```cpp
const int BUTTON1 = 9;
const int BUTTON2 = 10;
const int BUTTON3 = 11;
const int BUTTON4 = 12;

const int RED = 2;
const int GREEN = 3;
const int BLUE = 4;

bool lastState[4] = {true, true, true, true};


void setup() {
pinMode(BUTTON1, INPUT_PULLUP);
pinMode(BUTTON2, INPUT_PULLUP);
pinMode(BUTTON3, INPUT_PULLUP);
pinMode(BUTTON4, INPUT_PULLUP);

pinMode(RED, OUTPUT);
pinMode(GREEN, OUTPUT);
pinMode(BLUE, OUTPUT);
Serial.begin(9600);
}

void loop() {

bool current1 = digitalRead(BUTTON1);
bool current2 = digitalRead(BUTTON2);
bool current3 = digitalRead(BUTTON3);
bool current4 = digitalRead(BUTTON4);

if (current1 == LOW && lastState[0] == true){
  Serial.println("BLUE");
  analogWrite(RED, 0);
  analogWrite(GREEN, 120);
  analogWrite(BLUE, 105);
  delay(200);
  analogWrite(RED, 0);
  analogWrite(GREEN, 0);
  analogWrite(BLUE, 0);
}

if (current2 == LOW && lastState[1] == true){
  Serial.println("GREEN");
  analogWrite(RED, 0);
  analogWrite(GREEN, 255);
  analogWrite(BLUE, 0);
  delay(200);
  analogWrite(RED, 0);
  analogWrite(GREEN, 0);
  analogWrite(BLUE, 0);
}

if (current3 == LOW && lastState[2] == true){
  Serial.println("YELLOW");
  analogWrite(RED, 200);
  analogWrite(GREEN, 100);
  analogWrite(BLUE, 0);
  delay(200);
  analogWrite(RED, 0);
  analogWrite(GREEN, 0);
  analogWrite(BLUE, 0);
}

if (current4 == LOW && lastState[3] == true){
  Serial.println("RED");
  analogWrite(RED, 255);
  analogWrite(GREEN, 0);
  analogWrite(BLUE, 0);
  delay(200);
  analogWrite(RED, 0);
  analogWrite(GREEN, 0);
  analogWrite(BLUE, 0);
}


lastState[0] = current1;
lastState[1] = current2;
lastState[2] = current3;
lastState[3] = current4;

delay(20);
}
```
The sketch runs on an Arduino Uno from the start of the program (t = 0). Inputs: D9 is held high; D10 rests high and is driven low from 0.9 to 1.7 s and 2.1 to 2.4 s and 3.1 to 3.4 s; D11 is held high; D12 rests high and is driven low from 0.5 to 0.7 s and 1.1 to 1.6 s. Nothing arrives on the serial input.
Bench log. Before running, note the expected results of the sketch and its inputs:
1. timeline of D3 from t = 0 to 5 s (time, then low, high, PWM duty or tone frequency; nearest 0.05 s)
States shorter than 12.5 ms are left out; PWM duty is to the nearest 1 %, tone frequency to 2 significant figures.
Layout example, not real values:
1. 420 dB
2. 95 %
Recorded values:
1. 0 s low; 0.9 s high; 1.1 s low; 2.1 s high; 2.3 s low; 3.1 s high; 3.3 s low
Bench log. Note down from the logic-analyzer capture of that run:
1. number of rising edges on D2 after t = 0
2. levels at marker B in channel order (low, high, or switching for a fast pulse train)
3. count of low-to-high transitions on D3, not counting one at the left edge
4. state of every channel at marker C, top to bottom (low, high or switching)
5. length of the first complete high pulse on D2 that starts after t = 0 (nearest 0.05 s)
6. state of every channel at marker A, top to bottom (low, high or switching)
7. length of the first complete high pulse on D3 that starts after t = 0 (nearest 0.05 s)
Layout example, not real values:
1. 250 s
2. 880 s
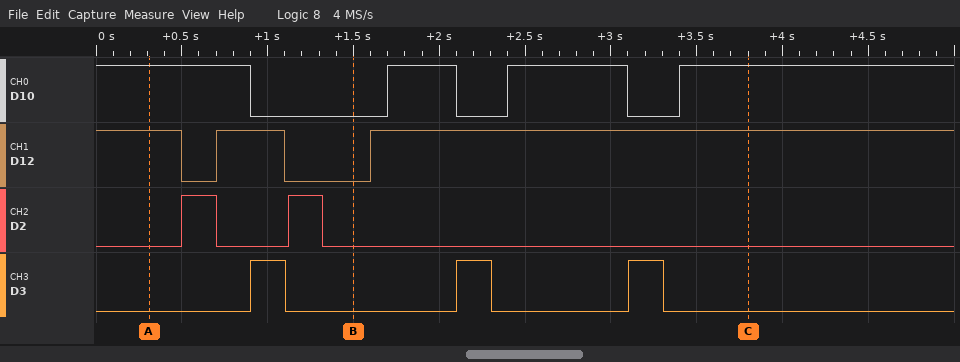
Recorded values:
1. 2
2. D10 low, D12 low, D2 low, D3 low
3. 3
4. D10 high, D12 high, D2 low, D3 low
5. 0.20 s
6. D10 high, D12 high, D2 low, D3 low
7. 0.20 s
